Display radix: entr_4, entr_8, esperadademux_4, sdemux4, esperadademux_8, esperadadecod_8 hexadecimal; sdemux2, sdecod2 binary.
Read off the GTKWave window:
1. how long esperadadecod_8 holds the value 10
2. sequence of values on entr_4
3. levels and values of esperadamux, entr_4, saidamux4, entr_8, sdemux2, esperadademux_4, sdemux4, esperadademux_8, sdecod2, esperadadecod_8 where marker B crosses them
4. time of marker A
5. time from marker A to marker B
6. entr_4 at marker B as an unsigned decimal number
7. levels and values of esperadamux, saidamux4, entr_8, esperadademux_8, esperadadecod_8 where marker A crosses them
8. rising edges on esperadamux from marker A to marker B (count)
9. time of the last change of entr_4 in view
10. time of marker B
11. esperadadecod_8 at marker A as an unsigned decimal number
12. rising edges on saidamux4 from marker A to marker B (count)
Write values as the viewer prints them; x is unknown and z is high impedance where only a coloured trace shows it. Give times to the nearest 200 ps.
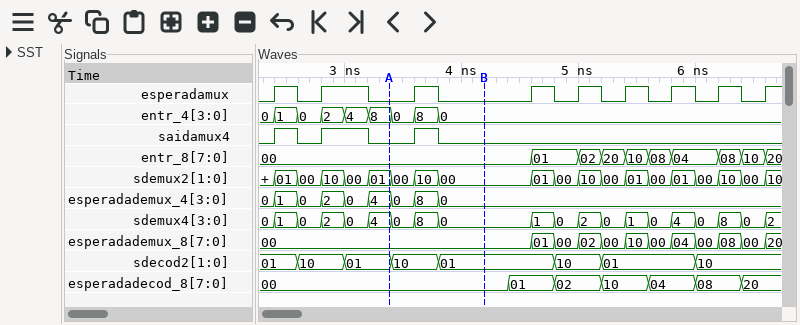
400 ps
0, 1, 0, 2, 4, 8, 0, 8, 0
esperadamux=0, entr_4=0, saidamux4=0, entr_8=00, sdemux2=00, esperadademux_4=0, sdemux4=0, esperadademux_8=00, sdecod2=01, esperadadecod_8=00
3400 ps
800 ps
0
esperadamux=0, saidamux4=0, entr_8=00, esperadademux_8=00, esperadadecod_8=00
1
3800 ps
4200 ps
0
1
